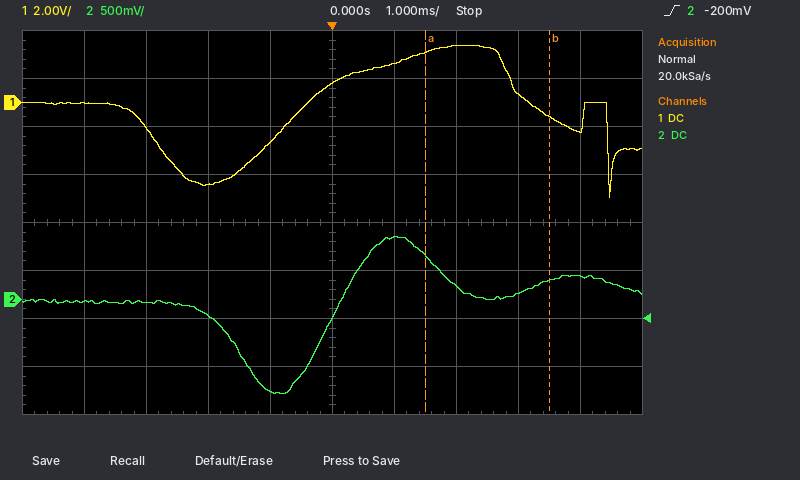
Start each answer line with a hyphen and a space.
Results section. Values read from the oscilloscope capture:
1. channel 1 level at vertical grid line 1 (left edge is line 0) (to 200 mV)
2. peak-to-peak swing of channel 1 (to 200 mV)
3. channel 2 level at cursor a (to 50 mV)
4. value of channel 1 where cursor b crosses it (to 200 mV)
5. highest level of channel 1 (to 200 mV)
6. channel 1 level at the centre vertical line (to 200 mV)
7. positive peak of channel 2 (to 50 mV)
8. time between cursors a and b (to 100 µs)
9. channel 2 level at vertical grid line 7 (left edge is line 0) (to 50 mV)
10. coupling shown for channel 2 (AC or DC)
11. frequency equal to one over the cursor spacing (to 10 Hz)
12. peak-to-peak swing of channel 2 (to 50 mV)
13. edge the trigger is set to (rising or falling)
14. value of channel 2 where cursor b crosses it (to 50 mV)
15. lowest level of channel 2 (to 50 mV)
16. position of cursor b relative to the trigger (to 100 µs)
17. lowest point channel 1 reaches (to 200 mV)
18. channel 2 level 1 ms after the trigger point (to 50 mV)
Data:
- 0.0 V
- 6.4 V
- 450 mV
- -600 mV
- 2.4 V
- 800 mV
- 650 mV
- 2.0 ms
- 150 mV
- DC
- 500 Hz
- 1.65 V
- rising
- 200 mV
- -1.00 V
- +3.5 ms
- -4.0 V
- 650 mV
